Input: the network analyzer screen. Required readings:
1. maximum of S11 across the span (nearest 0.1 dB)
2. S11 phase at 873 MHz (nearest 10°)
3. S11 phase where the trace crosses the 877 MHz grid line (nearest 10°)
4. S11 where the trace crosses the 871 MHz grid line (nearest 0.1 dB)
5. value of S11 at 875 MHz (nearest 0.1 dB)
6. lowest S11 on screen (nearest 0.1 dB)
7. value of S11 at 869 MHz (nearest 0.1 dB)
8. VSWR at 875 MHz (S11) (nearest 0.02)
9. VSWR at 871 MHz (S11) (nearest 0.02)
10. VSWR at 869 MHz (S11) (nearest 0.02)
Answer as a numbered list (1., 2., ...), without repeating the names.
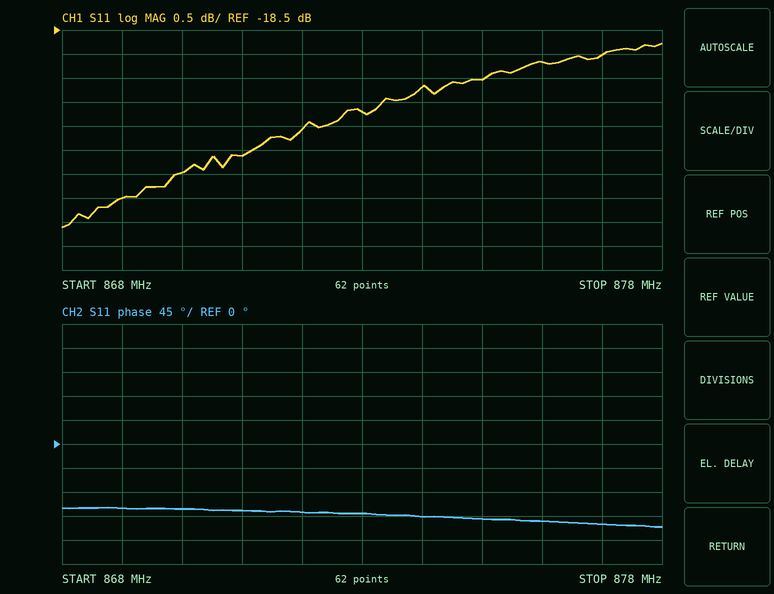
1. -18.8 dB
2. -130°
3. -150°
4. -21.1 dB
5. -19.5 dB
6. -22.6 dB
7. -22.0 dB
8. 1.24
9. 1.20
10. 1.18
